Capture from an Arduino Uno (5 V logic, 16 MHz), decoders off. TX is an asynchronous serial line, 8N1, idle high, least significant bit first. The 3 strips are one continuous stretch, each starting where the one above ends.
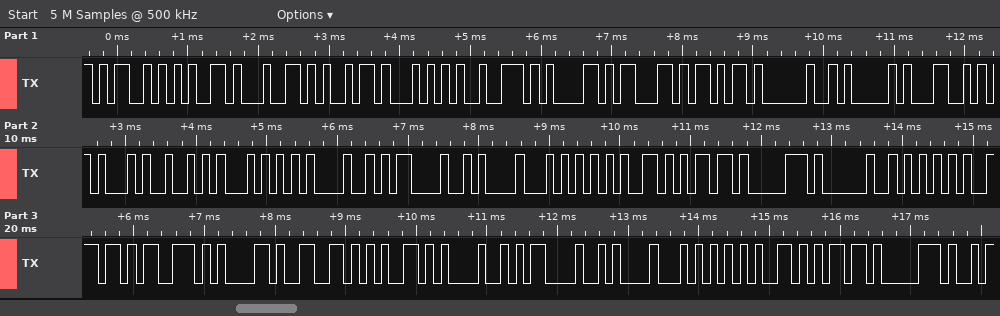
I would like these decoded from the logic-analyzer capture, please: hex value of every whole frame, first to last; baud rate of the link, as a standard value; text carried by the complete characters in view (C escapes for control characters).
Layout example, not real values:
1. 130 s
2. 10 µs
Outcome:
1. 4D 65 64 69 54 72 61 63 6B 20 41 4C 45 52 54 21 0D 0A 54 65 6D 70 20 55 6E 73 61 66 65 21 0D 0A 54 65 6D 70
2. 9600 baud
3. "MediTrack ALERT!\r\nTemp Unsafe!\r\nTemp"
